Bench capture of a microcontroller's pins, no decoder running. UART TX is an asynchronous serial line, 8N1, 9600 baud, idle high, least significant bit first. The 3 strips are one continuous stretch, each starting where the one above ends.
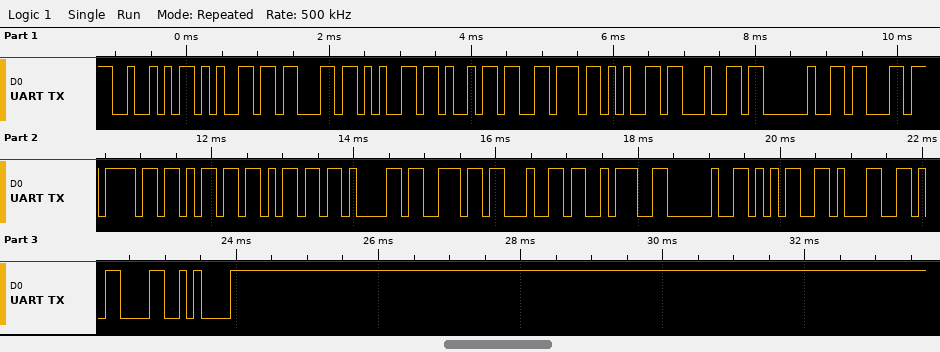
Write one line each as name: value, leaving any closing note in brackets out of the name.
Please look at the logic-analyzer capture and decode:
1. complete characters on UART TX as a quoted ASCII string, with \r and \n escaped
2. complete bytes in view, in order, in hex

complete characters on UART TX as a quoted ASCII string, with \r and \n escaped: "Received command: 51\r\n"
complete bytes in view, in order, in hex: 52 65 63 65 69 76 65 64 20 63 6F 6D 6D 61 6E 64 3A 20 35 31 0D 0A
